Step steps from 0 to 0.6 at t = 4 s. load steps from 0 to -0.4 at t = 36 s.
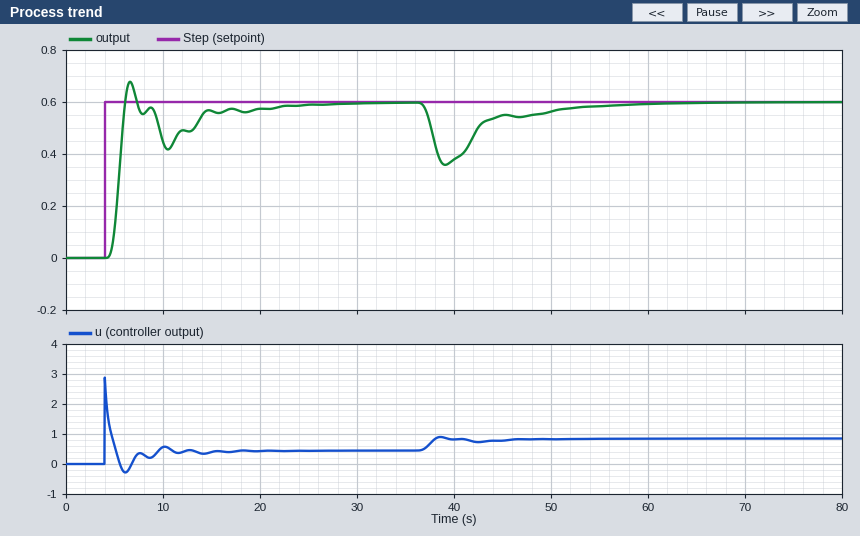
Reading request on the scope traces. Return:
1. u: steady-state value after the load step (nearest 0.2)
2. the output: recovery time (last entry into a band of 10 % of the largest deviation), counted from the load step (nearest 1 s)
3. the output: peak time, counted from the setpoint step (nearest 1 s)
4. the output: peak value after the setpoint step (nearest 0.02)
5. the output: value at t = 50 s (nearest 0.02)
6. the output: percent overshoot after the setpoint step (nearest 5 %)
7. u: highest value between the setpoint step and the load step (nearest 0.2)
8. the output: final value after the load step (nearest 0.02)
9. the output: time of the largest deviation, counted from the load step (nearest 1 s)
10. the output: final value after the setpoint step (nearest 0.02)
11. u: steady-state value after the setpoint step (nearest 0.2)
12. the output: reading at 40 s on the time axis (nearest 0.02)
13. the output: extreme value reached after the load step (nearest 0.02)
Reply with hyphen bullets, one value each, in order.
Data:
- 0.8
- 16 s
- 3 s
- 0.68
- 0.56
- 15 %
- 2.8
- 0.60
- 3 s
- 0.60
- 0.4
- 0.38
- 0.36
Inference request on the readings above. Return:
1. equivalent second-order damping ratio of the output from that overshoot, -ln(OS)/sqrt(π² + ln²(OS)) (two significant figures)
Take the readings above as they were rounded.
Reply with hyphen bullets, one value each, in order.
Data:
- 0.52
